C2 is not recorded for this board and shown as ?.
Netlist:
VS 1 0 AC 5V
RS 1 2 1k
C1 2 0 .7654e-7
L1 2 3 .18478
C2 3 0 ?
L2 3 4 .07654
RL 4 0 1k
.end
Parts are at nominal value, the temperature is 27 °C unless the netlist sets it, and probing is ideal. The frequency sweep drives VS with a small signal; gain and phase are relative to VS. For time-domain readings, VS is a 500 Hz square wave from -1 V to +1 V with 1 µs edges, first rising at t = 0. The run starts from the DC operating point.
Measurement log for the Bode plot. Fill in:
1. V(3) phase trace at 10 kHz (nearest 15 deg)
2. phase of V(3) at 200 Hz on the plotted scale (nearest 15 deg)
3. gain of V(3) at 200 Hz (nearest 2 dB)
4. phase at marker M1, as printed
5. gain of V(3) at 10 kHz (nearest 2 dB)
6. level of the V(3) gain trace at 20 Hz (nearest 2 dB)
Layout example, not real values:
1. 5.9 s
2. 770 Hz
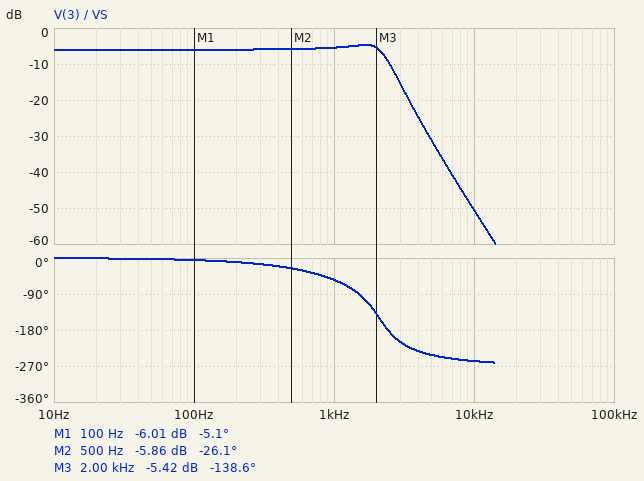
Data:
1. -255 deg
2. -15 deg
3. -6 dB
4. -5.1 deg
5. -50 dB
6. -6 dB
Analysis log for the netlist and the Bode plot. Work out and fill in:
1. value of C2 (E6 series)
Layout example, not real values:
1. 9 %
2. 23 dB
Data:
1. 100 nF
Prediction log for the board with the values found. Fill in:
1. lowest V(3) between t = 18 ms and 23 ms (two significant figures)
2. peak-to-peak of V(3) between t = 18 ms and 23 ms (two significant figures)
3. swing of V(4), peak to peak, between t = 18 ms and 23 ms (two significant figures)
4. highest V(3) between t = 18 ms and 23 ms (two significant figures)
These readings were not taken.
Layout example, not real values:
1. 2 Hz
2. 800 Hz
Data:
1. -680 mV
2. 1.4 V
3. 1.2 V
4. 680 mV
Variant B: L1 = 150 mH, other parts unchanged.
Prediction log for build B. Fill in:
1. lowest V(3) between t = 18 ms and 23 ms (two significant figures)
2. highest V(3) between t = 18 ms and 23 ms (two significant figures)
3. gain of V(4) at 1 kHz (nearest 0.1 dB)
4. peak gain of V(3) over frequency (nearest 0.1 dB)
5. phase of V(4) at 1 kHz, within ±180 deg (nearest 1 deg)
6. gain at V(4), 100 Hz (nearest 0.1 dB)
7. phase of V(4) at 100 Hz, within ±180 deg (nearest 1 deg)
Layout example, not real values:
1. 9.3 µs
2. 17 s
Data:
1. -720 mV
2. 720 mV
3. -6.2 dB
4. -3.9 dB
5. -74 deg
6. -6.0 dB
7. -7 deg
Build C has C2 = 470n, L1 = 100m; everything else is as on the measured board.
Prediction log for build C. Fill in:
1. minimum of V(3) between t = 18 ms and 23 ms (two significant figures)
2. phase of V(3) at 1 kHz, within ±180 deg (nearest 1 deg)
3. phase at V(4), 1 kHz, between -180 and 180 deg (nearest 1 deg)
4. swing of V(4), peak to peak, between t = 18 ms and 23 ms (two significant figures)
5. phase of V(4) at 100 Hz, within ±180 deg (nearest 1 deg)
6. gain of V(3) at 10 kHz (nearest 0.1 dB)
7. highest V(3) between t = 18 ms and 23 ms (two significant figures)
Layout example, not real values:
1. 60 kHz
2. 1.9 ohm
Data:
1. -490 mV
2. -91 deg
3. -117 deg
4. 980 mV
5. -13 deg
6. -58.8 dB
7. 490 mV
